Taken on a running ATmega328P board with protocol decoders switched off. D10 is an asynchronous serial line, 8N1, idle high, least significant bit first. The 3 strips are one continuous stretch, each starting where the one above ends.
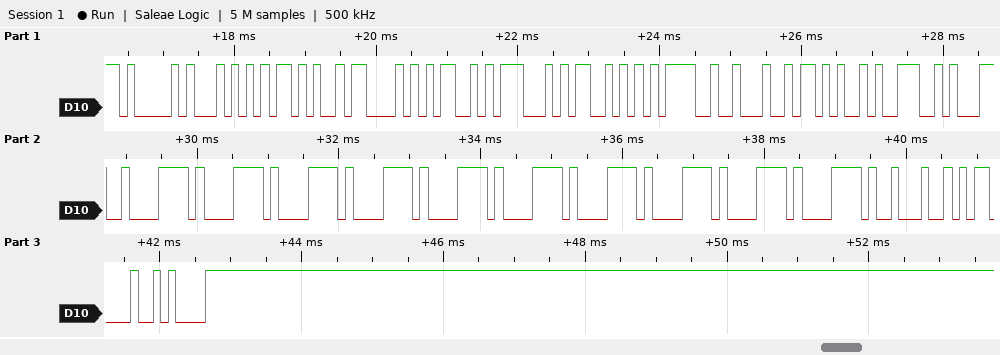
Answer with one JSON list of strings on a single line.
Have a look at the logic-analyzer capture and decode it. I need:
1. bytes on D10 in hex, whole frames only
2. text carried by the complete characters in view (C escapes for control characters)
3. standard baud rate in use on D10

["41 54 2B 43 4D 47 53 3D 22 2B 39 31 78 78 78 78 78 78 78 78 78 78 22 0D 0A", "\"AT+CMGS=\\\"+91xxxxxxxxxx\\\"\\r\\n\"", "9600 baud"]
